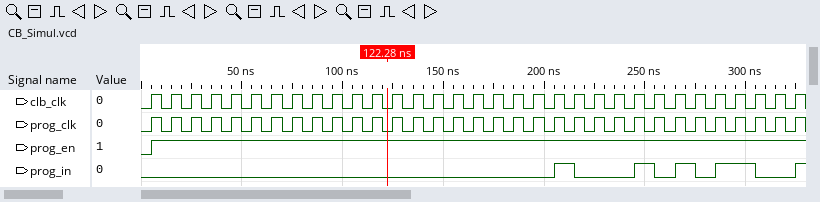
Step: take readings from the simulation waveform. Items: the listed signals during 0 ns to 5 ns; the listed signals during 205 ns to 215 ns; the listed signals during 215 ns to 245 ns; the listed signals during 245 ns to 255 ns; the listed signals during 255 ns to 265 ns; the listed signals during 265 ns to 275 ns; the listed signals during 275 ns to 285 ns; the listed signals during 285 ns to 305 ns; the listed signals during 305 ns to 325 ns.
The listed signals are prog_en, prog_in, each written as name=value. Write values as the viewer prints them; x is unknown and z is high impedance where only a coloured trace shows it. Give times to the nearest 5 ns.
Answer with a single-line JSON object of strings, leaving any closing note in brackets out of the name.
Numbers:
{"the listed signals during 0 ns to 5 ns": "prog_en=0, prog_in=0", "the listed signals during 205 ns to 215 ns": "prog_en=1, prog_in=1", "the listed signals during 215 ns to 245 ns": "prog_en=1, prog_in=0", "the listed signals during 245 ns to 255 ns": "prog_en=1, prog_in=1", "the listed signals during 255 ns to 265 ns": "prog_en=1, prog_in=0", "the listed signals during 265 ns to 275 ns": "prog_en=1, prog_in=1", "the listed signals during 275 ns to 285 ns": "prog_en=1, prog_in=0", "the listed signals during 285 ns to 305 ns": "prog_en=1, prog_in=1", "the listed signals during 305 ns to 325 ns": "prog_en=1, prog_in=0"}
